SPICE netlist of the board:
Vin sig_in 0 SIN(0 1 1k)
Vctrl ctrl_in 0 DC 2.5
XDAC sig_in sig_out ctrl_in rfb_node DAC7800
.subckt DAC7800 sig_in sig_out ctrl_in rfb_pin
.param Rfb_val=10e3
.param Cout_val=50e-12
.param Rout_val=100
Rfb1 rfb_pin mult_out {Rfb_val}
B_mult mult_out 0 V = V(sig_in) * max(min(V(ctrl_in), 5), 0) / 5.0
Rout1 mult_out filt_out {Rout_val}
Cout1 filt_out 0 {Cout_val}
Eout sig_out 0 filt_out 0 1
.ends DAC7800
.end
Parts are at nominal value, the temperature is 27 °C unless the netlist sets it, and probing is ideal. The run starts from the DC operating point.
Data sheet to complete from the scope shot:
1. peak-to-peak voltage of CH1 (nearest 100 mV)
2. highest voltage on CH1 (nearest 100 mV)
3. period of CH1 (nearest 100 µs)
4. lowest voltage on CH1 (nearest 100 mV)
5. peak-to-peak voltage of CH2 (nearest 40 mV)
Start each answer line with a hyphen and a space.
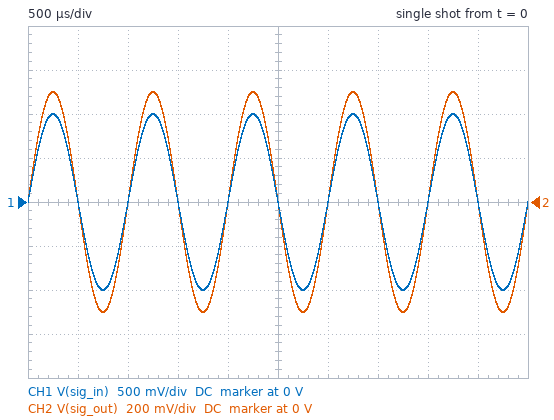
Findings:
- 2.0 V
- 1.0 V
- 1.0 ms
- -1.0 V
- 1.00 V
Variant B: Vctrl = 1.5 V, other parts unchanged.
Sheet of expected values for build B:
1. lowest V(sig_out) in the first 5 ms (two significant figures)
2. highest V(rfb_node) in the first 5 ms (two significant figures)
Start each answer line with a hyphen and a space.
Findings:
- -300 mV
- 300 mV
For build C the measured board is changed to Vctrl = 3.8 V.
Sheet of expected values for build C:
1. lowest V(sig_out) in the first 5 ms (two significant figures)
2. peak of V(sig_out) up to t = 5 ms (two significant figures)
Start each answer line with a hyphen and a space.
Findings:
- -760 mV
- 760 mV
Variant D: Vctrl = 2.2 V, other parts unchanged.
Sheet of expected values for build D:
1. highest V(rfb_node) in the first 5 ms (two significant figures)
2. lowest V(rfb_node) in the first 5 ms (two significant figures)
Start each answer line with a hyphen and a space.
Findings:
- 440 mV
- -440 mV
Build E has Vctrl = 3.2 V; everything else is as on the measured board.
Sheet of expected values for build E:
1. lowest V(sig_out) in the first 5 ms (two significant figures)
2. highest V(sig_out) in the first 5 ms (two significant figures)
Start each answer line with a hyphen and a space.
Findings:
- -640 mV
- 640 mV
